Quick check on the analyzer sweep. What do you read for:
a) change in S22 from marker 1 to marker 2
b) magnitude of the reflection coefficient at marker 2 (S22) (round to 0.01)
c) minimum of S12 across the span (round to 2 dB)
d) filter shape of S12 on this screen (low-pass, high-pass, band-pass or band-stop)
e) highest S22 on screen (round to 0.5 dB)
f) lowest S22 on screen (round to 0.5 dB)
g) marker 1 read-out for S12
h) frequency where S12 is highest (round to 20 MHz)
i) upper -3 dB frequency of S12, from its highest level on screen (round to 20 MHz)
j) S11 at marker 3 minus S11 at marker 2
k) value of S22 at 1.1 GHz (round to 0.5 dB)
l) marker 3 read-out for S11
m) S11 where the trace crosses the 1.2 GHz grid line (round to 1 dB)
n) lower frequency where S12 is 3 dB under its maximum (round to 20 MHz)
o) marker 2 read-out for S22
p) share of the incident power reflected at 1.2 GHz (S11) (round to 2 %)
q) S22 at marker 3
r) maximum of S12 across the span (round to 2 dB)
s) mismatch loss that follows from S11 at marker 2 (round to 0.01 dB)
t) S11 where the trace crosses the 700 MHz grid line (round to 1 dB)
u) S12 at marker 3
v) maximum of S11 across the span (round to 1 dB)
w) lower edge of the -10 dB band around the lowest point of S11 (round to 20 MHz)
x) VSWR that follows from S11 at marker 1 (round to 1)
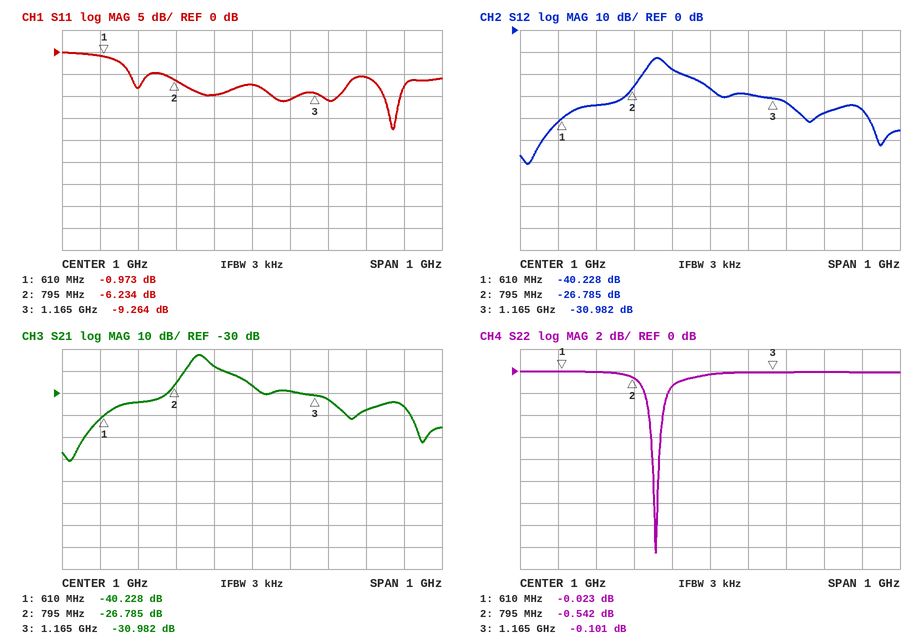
-0.519 dB
0.94
-60 dB
band-pass
0.0 dB
-16.5 dB
-40.228 dB
860 MHz
880 MHz
-3.030 dB
0.0 dB
-9.264 dB
-11 dB
840 MHz
-0.542 dB
8 %
-0.101 dB
-12 dB
1.18 dB
-8 dB
-30.982 dB
0 dB
1.34 GHz
18
